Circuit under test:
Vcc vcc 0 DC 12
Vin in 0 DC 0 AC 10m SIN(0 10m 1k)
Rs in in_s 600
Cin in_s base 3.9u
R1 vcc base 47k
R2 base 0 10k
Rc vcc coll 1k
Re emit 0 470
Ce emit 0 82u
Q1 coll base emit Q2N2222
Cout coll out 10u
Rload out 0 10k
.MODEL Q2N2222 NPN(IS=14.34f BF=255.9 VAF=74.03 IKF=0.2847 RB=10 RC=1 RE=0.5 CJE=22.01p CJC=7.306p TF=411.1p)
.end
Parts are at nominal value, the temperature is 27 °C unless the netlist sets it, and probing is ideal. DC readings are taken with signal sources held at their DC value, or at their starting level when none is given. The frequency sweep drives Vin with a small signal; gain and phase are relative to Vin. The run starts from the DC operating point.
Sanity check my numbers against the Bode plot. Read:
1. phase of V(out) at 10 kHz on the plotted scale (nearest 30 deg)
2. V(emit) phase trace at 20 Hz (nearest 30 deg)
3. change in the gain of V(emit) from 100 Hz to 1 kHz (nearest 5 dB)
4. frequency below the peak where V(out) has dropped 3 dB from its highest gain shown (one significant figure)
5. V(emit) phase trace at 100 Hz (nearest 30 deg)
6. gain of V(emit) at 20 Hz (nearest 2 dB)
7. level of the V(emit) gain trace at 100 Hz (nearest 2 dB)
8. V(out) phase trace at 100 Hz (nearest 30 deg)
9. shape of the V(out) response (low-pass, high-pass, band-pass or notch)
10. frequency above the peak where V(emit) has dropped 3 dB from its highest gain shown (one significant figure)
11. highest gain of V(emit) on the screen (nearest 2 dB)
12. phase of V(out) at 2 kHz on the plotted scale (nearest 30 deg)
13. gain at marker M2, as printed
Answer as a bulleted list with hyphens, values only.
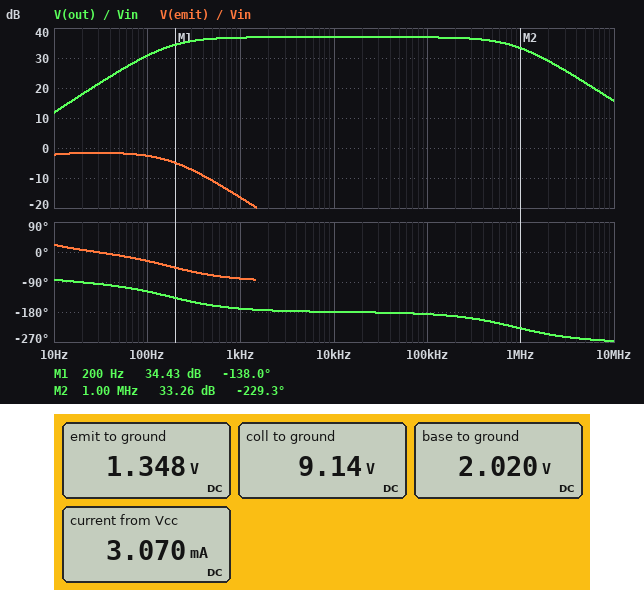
- -180 deg
- 0 deg
- -15 dB
- 200 Hz
- -30 deg
- -2 dB
- -2 dB
- -120 deg
- band-pass
- 200 Hz
- -2 dB
- -180 deg
- 33.26 dB
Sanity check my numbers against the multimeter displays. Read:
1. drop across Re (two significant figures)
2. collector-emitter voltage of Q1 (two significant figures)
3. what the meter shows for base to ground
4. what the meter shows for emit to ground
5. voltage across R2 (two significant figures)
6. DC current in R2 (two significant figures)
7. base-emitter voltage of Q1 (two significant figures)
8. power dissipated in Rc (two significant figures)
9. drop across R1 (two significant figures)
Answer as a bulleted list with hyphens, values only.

- 1.3 V
- 7.8 V
- 2.020 V
- 1.348 V
- 2.0 V
- 200 µA
- 670 mV
- 8.2 mW
- 10 V
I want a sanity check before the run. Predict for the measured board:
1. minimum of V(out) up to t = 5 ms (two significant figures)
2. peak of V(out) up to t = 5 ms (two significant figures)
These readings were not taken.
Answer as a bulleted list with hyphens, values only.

- -720 mV
- 680 mV
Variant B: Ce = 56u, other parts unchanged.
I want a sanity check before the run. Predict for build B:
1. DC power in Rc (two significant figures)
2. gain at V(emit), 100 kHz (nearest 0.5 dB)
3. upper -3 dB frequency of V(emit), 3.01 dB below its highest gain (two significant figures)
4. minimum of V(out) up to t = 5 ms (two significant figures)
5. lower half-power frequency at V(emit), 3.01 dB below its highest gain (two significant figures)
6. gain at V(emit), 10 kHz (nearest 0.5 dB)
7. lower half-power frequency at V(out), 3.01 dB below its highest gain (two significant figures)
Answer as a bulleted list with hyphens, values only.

- 8.2 mW
- -53.0 dB
- 260 Hz
- -710 mV
- 4.5 Hz
- -33.0 dB
- 250 Hz
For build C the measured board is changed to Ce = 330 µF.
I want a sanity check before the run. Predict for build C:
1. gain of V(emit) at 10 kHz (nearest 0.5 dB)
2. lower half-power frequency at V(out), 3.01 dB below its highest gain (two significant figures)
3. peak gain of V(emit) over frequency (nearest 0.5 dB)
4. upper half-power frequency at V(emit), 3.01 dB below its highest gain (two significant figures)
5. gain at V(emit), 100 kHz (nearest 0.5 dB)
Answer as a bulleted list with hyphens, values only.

- -48.5 dB
- 53 Hz
- -3.5 dB
- 60 Hz
- -68.5 dB
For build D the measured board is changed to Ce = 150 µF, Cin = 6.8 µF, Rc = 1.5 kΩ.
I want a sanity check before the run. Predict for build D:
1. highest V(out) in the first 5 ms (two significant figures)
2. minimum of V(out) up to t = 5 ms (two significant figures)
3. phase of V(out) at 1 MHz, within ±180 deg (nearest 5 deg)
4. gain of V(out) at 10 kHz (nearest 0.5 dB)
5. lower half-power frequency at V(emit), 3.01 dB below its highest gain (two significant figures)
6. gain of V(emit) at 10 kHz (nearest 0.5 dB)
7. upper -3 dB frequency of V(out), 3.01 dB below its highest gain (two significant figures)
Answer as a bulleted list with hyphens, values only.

- 960 mV
- -1.0 V
- 120 deg
- 40.0 dB
- 2.5 Hz
- -42.0 dB
- 620 kHz
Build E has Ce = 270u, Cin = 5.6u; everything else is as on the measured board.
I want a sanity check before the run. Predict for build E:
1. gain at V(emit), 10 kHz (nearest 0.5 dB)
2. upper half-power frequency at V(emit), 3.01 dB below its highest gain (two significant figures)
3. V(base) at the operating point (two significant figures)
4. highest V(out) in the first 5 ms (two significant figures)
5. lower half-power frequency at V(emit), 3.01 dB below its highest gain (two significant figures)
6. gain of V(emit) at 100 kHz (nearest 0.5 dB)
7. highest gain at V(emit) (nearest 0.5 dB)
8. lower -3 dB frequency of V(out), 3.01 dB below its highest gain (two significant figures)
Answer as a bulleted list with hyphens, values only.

- -47.0 dB
- 64 Hz
- 2.0 V
- 670 mV
- 2.7 Hz
- -67.0 dB
- -2.5 dB
- 58 Hz
